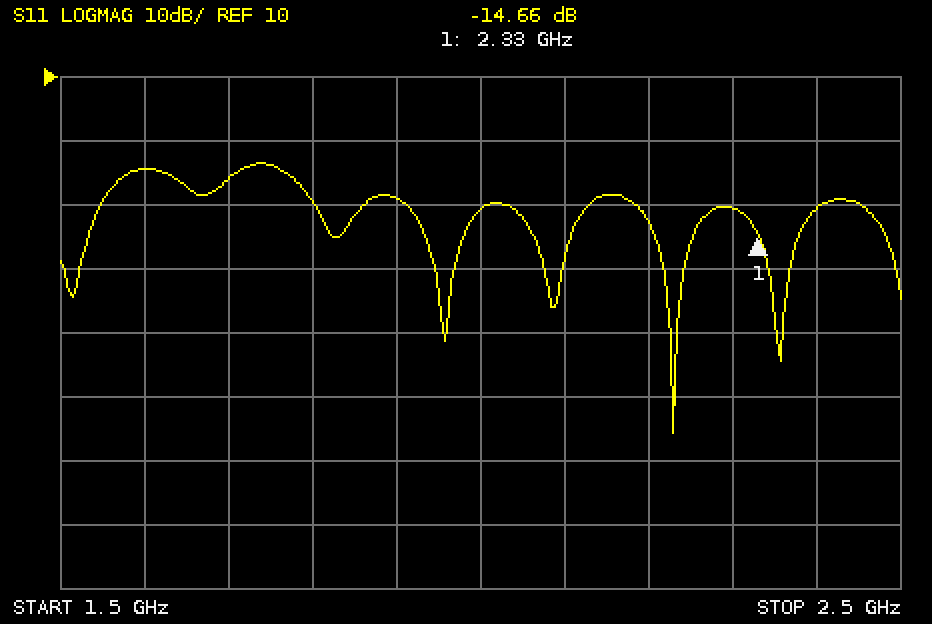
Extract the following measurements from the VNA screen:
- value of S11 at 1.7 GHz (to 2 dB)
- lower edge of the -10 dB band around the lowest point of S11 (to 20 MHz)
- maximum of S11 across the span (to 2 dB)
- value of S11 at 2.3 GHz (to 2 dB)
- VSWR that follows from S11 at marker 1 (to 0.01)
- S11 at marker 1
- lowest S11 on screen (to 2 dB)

-6 dB
2.18 GHz
-4 dB
-10 dB
1.45
-14.66 dB
-46 dB
